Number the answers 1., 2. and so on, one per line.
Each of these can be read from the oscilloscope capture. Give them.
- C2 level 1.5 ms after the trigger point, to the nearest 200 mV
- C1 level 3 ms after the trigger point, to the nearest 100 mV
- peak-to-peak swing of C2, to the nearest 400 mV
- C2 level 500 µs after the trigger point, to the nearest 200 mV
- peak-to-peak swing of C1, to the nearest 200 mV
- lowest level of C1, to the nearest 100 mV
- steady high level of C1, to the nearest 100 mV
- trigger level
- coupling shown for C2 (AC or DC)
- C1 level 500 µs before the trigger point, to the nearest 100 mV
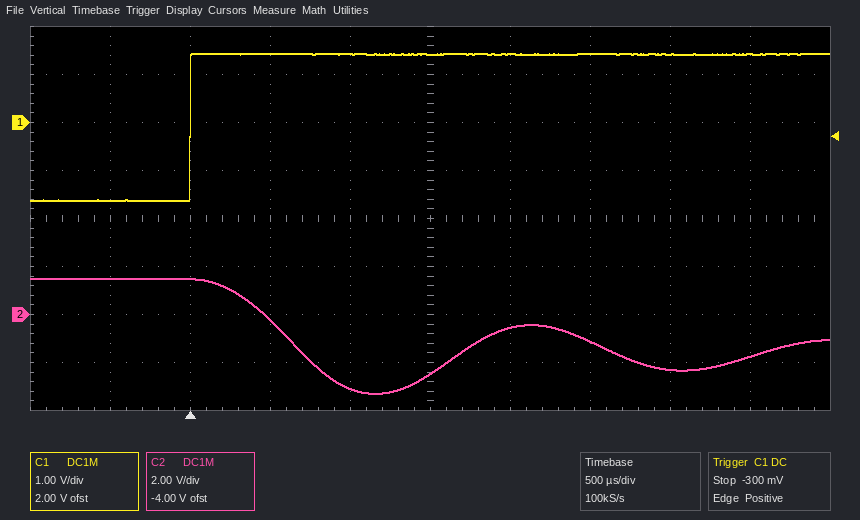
1. -2.4 V
2. 1.4 V
3. 4.8 V
4. -200 mV
5. 3.0 V
6. -1.6 V
7. 1.4 V
8. -300 mV
9. DC
10. -1.6 V
